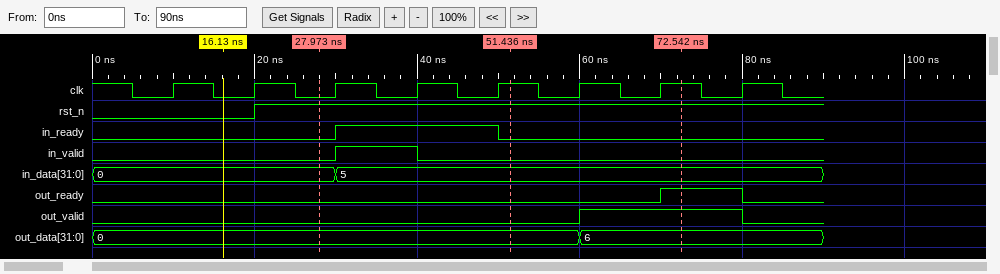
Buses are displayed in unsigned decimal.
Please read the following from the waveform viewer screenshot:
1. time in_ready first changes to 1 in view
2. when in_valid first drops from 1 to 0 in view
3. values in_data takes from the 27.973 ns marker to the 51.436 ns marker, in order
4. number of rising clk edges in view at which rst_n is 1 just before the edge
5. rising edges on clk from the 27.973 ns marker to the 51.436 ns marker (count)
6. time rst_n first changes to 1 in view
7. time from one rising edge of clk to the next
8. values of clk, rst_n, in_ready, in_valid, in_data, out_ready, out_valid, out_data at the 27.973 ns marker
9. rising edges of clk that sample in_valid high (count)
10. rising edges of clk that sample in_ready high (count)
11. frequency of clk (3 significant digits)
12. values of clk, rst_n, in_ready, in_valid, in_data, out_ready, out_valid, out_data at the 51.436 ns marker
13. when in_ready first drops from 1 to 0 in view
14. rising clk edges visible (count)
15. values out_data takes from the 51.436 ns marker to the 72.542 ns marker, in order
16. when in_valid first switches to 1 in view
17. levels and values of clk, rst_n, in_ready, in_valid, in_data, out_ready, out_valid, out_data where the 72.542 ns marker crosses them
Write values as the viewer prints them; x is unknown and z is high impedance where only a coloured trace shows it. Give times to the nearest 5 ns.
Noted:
30 ns
40 ns
0, 5
6
3
20 ns
10 ns
clk=0, rst_n=1, in_ready=0, in_valid=0, in_data=0, out_ready=0, out_valid=0, out_data=0
1
2
100 MHz
clk=1, rst_n=1, in_ready=0, in_valid=0, in_data=5, out_ready=0, out_valid=0, out_data=0
50 ns
8
0, 6
30 ns
clk=1, rst_n=1, in_ready=0, in_valid=0, in_data=5, out_ready=1, out_valid=1, out_data=6
